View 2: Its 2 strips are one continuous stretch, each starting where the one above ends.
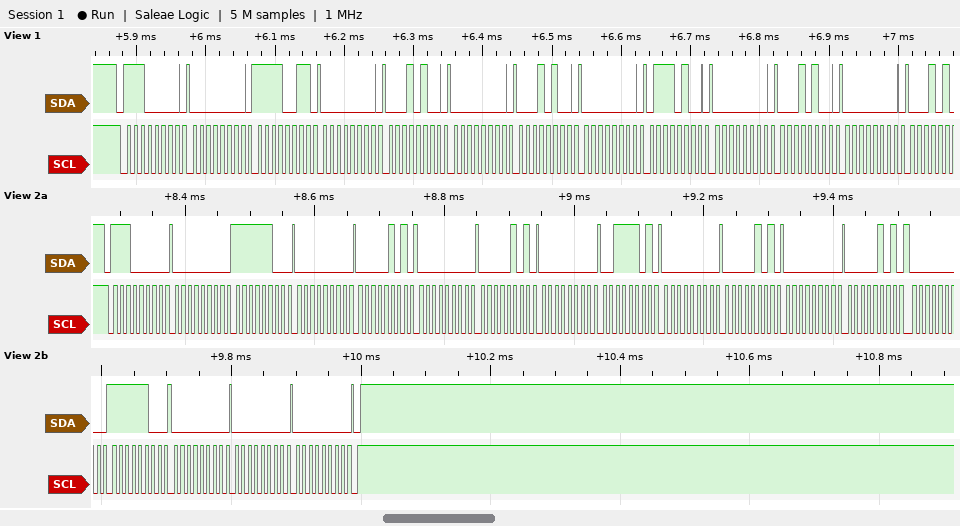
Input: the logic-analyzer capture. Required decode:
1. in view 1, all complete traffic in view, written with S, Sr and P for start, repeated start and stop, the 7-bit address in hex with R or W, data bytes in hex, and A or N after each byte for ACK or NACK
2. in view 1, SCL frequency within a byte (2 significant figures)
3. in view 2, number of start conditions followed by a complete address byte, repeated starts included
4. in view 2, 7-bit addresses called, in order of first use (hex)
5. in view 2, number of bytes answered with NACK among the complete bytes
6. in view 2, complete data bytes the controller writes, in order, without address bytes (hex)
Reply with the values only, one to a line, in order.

S 70W A 00 A F3 A 00 A 14 A 00 A 14 A 00 A 74 A 00 A 14 A 00 A
100 kHz
1
0x70
0
00 FC 00 05 00 05 00 3D 00 05 00 05 00 FC 00 00 00
